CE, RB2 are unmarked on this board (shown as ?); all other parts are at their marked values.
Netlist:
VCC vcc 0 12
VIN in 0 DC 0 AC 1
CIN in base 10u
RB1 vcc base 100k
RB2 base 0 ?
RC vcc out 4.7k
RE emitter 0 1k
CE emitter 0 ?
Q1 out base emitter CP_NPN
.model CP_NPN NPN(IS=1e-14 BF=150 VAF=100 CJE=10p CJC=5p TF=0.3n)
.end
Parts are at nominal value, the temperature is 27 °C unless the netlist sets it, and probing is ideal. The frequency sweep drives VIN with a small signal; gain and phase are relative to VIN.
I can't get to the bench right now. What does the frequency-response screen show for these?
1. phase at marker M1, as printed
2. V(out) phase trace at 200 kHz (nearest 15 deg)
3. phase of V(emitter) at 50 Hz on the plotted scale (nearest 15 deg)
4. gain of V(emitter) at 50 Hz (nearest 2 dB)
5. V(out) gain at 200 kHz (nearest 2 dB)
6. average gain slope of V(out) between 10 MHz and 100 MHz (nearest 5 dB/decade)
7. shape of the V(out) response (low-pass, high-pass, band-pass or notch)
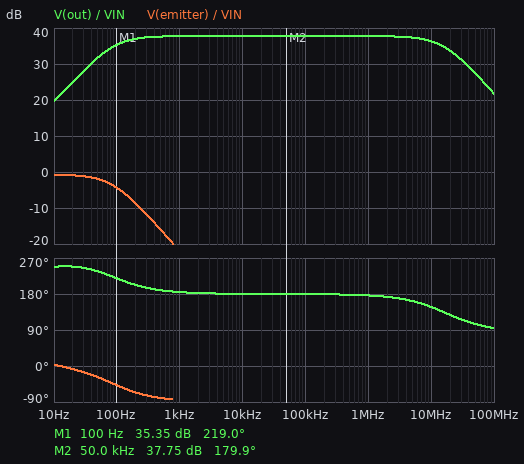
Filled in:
219.0 deg
180 deg
-30 deg
-2 dB
38 dB
-15 dB/decade
band-pass
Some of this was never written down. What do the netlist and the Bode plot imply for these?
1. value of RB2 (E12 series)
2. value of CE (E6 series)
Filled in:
10 kΩ
33 µF
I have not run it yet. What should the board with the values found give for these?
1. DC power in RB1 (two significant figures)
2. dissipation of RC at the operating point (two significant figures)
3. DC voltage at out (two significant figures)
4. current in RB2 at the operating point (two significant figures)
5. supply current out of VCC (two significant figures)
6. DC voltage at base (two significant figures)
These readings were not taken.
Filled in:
1.2 mW
880 µW
10 V
110 µA
540 µA
1.1 V
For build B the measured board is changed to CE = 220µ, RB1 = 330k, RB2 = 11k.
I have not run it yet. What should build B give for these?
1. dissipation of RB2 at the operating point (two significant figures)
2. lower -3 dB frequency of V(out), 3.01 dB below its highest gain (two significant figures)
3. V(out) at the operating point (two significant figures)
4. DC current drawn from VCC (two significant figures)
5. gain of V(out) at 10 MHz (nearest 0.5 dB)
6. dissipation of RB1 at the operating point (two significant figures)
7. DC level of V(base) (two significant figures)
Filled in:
14 µW
17 MHz
12 V
35 µA
-6.0 dB
410 µW
390 mV
